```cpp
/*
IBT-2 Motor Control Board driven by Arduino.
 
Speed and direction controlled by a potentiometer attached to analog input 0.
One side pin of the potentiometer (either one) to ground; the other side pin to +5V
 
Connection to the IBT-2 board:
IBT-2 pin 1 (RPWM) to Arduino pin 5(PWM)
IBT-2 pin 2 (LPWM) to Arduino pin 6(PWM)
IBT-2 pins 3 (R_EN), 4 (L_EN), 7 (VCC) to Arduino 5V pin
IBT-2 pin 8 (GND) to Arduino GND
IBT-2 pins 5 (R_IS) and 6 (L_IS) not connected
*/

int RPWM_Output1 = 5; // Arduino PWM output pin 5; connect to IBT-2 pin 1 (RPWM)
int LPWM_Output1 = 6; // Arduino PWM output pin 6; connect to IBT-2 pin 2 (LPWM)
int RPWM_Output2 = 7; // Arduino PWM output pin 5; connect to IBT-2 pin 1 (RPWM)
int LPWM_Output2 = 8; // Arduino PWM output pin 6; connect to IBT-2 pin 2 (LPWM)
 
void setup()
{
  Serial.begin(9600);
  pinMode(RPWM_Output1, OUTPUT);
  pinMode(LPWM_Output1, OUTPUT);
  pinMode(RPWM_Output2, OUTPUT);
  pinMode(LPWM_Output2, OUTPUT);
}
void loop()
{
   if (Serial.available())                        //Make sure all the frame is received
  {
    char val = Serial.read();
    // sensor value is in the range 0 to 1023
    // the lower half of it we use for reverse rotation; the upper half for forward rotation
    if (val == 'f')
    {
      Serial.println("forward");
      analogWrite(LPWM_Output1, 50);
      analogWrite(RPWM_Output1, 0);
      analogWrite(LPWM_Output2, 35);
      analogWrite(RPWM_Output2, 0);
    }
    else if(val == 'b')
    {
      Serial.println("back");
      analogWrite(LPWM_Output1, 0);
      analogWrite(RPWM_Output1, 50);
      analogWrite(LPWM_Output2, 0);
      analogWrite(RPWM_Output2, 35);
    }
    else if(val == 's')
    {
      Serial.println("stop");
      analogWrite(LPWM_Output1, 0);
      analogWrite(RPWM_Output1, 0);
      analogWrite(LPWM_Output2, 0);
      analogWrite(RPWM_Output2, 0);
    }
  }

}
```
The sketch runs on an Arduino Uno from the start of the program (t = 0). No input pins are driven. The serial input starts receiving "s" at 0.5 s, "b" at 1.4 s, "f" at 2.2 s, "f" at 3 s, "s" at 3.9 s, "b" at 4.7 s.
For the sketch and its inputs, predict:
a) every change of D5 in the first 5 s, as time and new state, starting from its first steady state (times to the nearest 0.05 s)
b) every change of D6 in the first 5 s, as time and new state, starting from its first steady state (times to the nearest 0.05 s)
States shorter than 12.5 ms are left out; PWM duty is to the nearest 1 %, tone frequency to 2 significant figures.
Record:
0 s low; 1.4 s PWM 20 %; 2.2 s low; 4.7 s PWM 20 %
0 s low; 2.2 s PWM 20 %; 3.9 s low
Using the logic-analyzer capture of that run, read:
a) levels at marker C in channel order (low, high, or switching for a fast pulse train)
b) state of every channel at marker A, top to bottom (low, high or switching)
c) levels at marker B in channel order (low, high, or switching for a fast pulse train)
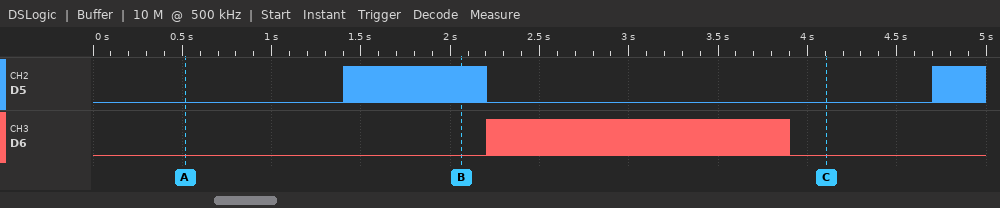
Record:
D5 low, D6 low
D5 low, D6 low
D5 switching, D6 low
